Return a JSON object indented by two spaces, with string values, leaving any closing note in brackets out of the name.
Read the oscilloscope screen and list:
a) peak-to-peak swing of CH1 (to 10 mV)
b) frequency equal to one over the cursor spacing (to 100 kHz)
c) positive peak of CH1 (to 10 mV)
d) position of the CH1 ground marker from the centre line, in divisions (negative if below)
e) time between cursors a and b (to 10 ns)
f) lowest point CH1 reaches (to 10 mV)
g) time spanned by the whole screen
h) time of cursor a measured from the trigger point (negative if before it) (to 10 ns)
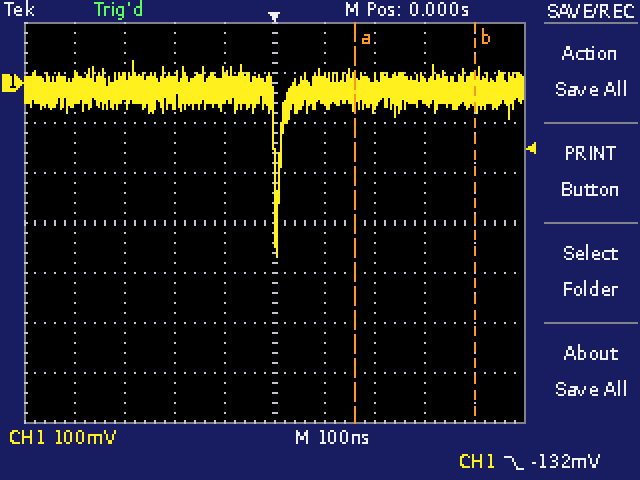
{
  "peak-to-peak swing of CH1": "390 mV",
  "frequency equal to one over the cursor spacing": "4.2 MHz",
  "positive peak of CH1": "40 mV",
  "position of the CH1 ground marker from the centre line, in divisions": "+2.8 div",
  "time between cursors a and b": "240 ns",
  "lowest point CH1 reaches": "-350 mV",
  "time spanned by the whole screen": "1 µs",
  "time of cursor a measured from the trigger point (negative if before it)": "+160 ns"
}
